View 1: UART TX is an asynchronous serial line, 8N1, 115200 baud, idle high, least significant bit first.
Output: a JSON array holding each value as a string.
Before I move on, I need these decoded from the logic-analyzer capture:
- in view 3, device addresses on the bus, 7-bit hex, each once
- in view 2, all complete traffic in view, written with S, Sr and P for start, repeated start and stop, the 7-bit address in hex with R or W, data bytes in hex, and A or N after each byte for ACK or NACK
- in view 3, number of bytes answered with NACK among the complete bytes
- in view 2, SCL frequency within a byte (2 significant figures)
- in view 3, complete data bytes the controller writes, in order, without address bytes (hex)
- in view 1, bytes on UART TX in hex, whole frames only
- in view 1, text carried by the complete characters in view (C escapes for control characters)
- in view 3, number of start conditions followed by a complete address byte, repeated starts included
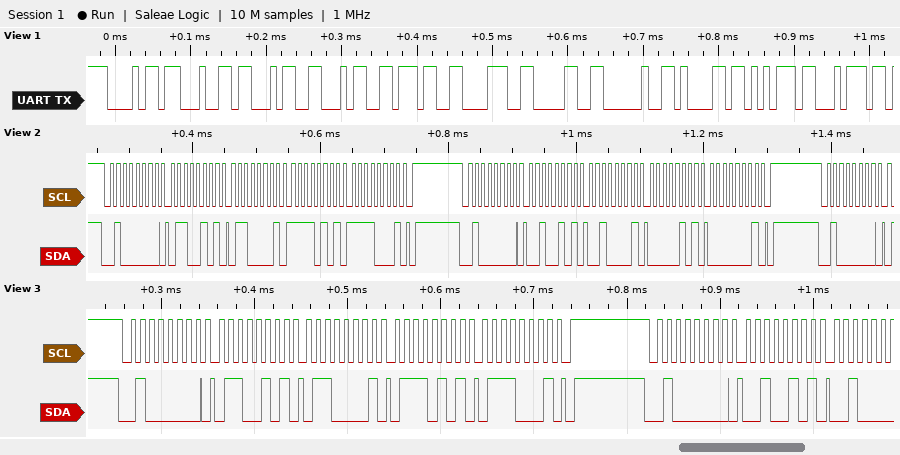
["0x20", "S 20W A 65 A 61 A F5 A F1 A P S 20W A 25 A 21 A 05 A 01 A P S 20W A", "0", "100 kHz", "65 61 75 71 25", "68 64 34 34 37 38 30 20 61 75 74", "\"hd44780 aut\"", "2"]
